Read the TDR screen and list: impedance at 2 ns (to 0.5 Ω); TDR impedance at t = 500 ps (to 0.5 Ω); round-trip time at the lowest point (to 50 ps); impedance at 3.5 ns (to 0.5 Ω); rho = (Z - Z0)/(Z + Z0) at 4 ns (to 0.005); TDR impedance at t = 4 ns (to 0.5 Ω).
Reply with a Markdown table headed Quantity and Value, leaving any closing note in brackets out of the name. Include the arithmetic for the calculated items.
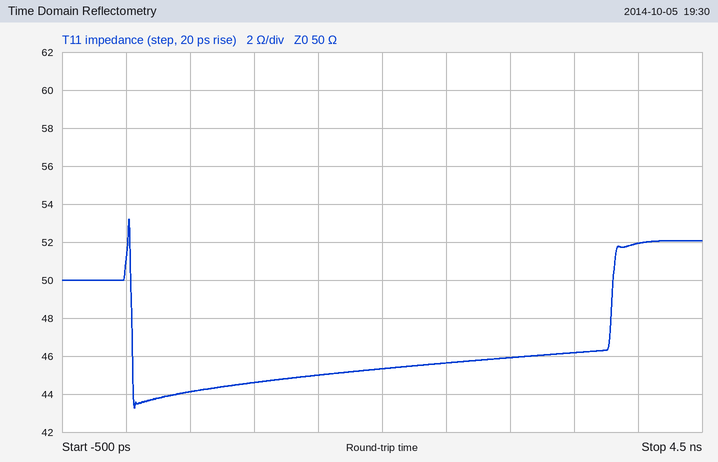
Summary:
| Quantity | Value |
|---|---|
| impedance at 2 ns | 45.5 Ω |
| TDR impedance at t = 500 ps | 44.0 Ω |
| round-trip time at the lowest point | 50 ps |
| impedance at 3.5 ns | 46.0 Ω |
| rho = (Z - Z0)/(Z + Z0) at 4 ns | (52 − 50)/(52 + 50) ≈ +0.020 |
| TDR impedance at t = 4 ns | 52.0 Ω |
